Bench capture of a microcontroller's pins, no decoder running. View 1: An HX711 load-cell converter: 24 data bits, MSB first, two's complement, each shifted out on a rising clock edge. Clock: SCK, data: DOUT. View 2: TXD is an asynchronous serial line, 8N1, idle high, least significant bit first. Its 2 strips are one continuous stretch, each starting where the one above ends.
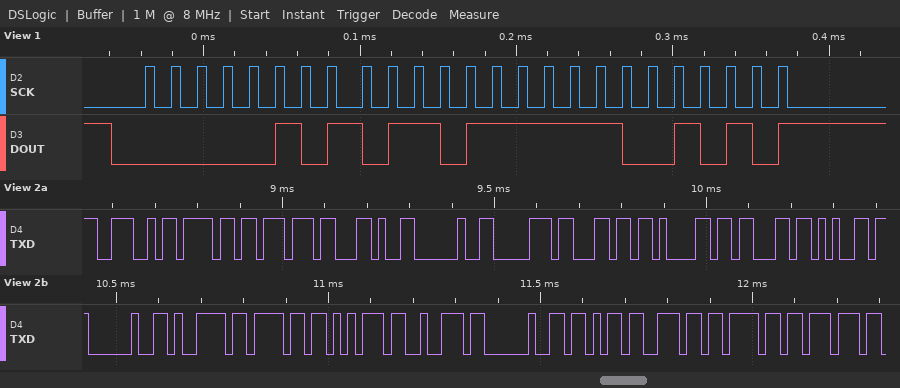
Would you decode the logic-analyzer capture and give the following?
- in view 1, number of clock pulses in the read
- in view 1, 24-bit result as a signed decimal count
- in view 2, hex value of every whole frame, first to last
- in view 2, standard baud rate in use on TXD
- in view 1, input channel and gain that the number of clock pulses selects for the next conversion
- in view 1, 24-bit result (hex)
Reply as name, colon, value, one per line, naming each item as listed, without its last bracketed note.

in view 1, number of clock pulses in the read: 25
in view 1, 24-bit result as a signed decimal count: 356298
in view 2, hex value of every whole frame, first to last: 0x4E 0x6F 0x77 0x2C 0x20 0x70 0x6C 0x61 0x63 0x65 0x20 0x79 0x6F 0x75 0x72 0x20 0x6B 0x6E 0x6F 0x77
in view 2, standard baud rate in use on TXD: 57600 baud
in view 1, input channel and gain that the number of clock pulses selects for the next conversion: channel A, gain 128
in view 1, 24-bit result: 0x056FCA
